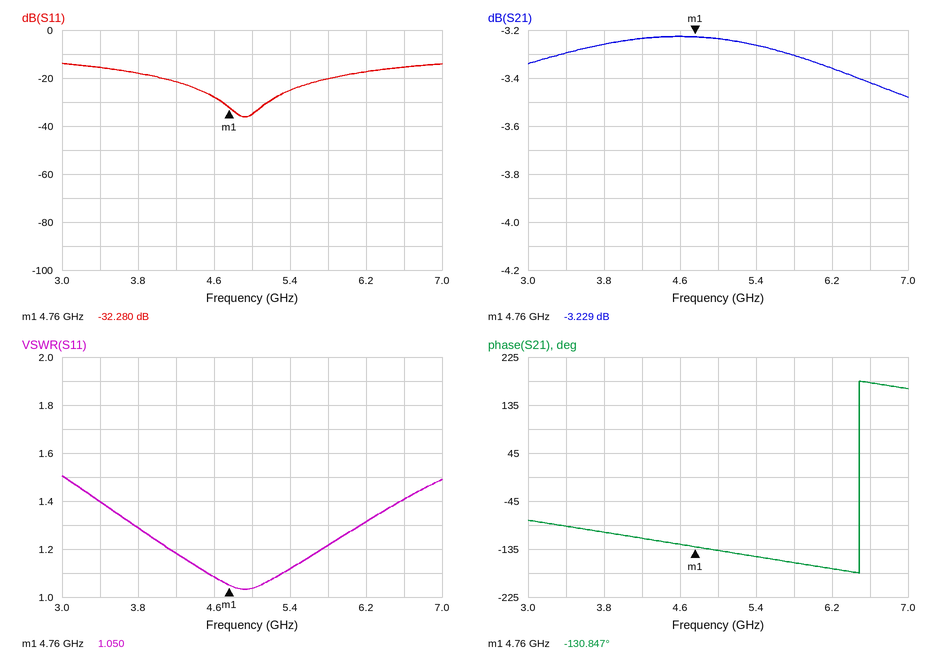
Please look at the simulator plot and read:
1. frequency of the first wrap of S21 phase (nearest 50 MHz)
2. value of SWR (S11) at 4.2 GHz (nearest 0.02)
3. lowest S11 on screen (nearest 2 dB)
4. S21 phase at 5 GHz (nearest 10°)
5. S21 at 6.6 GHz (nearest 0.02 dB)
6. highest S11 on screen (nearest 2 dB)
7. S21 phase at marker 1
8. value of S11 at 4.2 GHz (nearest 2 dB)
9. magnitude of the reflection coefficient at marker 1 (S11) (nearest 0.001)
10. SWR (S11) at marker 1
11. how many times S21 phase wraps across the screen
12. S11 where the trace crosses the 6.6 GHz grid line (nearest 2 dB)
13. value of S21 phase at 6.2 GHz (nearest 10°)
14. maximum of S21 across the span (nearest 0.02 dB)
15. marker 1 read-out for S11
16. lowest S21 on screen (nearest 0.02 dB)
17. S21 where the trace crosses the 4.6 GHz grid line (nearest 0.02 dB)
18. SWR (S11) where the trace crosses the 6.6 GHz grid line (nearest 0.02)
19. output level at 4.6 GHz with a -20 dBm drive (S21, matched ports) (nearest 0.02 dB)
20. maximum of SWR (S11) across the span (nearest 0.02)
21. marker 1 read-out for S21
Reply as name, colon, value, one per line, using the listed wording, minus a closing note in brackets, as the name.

frequency of the first wrap of S21 phase: 6.50 GHz
value of SWR (S11) at 4.2 GHz: 1.18
lowest S11 on screen: -36 dB
S21 phase at 5 GHz: -140°
S21 at 6.6 GHz: -3.42 dB
highest S11 on screen: -14 dB
S21 phase at marker 1: -130.847°
value of S11 at 4.2 GHz: -22 dB
magnitude of the reflection coefficient at marker 1 (S11): 0.024
SWR (S11) at marker 1: 1.050
how many times S21 phase wraps across the screen: 1
S11 where the trace crosses the 6.6 GHz grid line: -16 dB
value of S21 phase at 6.2 GHz: -170°
maximum of S21 across the span: -3.22 dB
marker 1 read-out for S11: -32.280 dB
lowest S21 on screen: -3.48 dB
S21 where the trace crosses the 4.6 GHz grid line: -3.22 dB
SWR (S11) where the trace crosses the 6.6 GHz grid line: 1.40
output level at 4.6 GHz with a -20 dBm drive (S21, matched ports): -23.22 dBm
maximum of SWR (S11) across the span: 1.50
marker 1 read-out for S21: -3.229 dB
